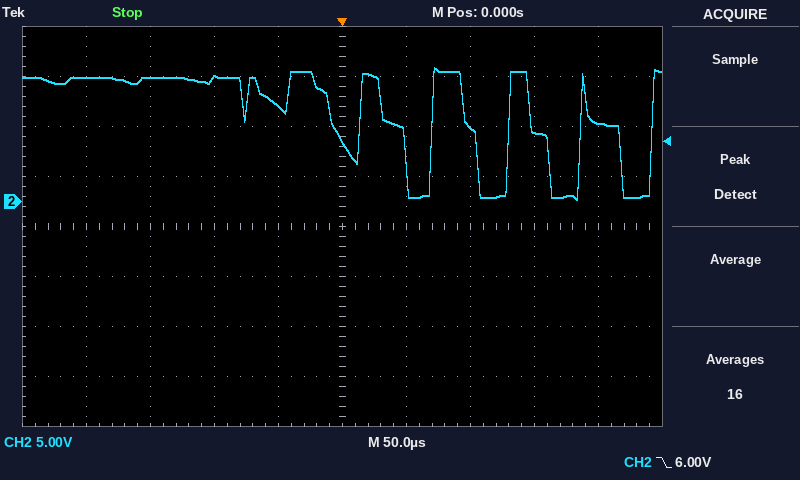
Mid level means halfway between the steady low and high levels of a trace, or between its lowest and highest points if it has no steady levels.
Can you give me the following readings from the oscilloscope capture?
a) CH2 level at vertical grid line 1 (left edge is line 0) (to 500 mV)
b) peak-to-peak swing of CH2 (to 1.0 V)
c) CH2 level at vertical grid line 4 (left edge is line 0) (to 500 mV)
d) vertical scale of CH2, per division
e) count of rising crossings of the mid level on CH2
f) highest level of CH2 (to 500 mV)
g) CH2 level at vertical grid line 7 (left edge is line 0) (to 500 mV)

12.5 V
13.0 V
9.5 V
5 V
5
13.5 V
7.5 V
